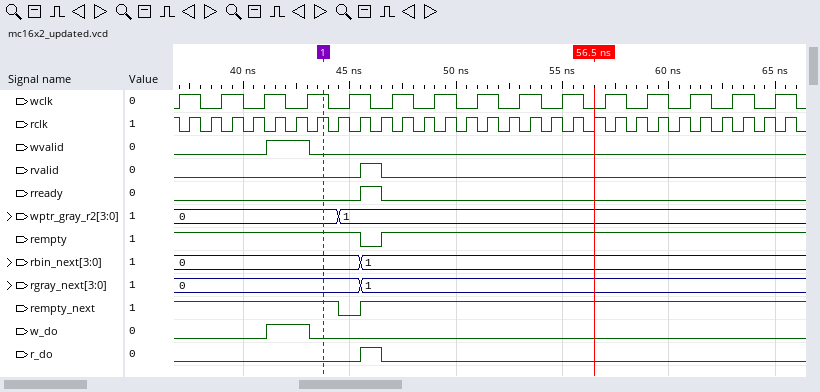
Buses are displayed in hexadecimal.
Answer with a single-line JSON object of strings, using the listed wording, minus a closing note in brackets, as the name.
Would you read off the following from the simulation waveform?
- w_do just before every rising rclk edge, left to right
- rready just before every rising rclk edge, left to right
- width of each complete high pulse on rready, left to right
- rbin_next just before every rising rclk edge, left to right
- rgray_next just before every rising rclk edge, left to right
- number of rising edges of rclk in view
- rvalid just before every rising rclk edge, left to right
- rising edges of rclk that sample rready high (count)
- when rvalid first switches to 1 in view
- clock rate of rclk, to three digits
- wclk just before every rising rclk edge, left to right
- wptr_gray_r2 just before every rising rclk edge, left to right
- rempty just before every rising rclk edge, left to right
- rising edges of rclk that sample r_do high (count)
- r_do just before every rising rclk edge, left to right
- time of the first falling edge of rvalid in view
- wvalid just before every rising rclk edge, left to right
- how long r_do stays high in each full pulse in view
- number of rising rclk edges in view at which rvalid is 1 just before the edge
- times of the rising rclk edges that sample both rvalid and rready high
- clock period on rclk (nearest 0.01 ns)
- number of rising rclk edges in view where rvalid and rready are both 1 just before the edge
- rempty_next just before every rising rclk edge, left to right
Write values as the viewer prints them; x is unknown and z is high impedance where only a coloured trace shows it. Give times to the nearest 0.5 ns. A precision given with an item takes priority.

{"w_do just before every rising rclk edge, left to right": "0 0 0 0 1 1 0 0 0 0 0 0 0 0 0 0 0 0 0 0 0 0 0 0 0 0 0 0 0", "rready just before every rising rclk edge, left to right": "0 0 0 0 0 0 0 0 0 1 0 0 0 0 0 0 0 0 0 0 0 0 0 0 0 0 0 0 0", "width of each complete high pulse on rready, left to right": "1 ns", "rbin_next just before every rising rclk edge, left to right": "0, 0, 0, 0, 0, 0, 0, 0, 0, 1, 1, 1, 1, 1, 1, 1, 1, 1, 1, 1, 1, 1, 1, 1, 1, 1, 1, 1, 1", "rgray_next just before every rising rclk edge, left to right": "0, 0, 0, 0, 0, 0, 0, 0, 0, 1, 1, 1, 1, 1, 1, 1, 1, 1, 1, 1, 1, 1, 1, 1, 1, 1, 1, 1, 1", "number of rising edges of rclk in view": "29", "rvalid just before every rising rclk edge, left to right": "0 0 0 0 0 0 0 0 0 1 0 0 0 0 0 0 0 0 0 0 0 0 0 0 0 0 0 0 0", "rising edges of rclk that sample rready high": "1", "when rvalid first switches to 1 in view": "45.5 ns", "clock rate of rclk, to three digits": "1.00 GHz", "wclk just before every rising rclk edge, left to right": "1 0 1 0 1 0 1 0 1 0 1 0 1 0 1 0 1 0 1 0 1 0 1 0 1 0 1 0 1", "wptr_gray_r2 just before every rising rclk edge, left to right": "0, 0, 0, 0, 0, 0, 0, 0, 1, 1, 1, 1, 1, 1, 1, 1, 1, 1, 1, 1, 1, 1, 1, 1, 1, 1, 1, 1, 1", "rempty just before every rising rclk edge, left to right": "1 1 1 1 1 1 1 1 1 0 1 1 1 1 1 1 1 1 1 1 1 1 1 1 1 1 1 1 1", "rising edges of rclk that sample r_do high": "1", "r_do just before every rising rclk edge, left to right": "0 0 0 0 0 0 0 0 0 1 0 0 0 0 0 0 0 0 0 0 0 0 0 0 0 0 0 0 0", "time of the first falling edge of rvalid in view": "46.5 ns", "wvalid just before every rising rclk edge, left to right": "0 0 0 0 1 1 0 0 0 0 0 0 0 0 0 0 0 0 0 0 0 0 0 0 0 0 0 0 0", "how long r_do stays high in each full pulse in view": "1 ns", "number of rising rclk edges in view at which rvalid is 1 just before the edge": "1", "times of the rising rclk edges that sample both rvalid and rready high": "46.5 ns", "clock period on rclk": "1 ns", "number of rising rclk edges in view where rvalid and rready are both 1 just before the edge": "1", "rempty_next just before every rising rclk edge, left to right": "1 1 1 1 1 1 1 1 0 1 1 1 1 1 1 1 1 1 1 1 1 1 1 1 1 1 1 1 1"}
